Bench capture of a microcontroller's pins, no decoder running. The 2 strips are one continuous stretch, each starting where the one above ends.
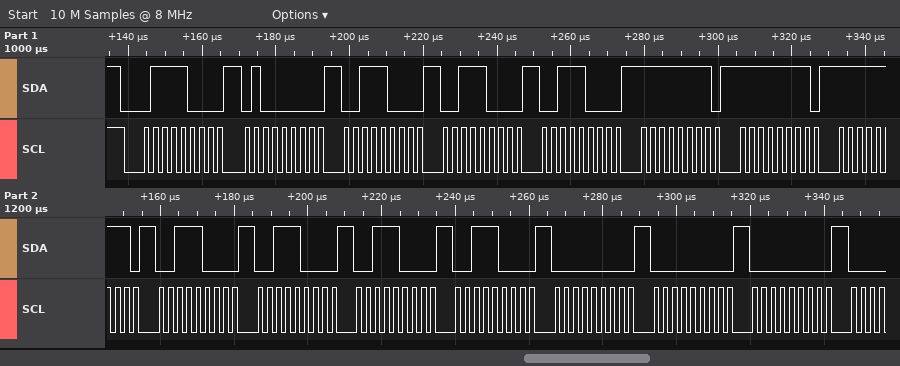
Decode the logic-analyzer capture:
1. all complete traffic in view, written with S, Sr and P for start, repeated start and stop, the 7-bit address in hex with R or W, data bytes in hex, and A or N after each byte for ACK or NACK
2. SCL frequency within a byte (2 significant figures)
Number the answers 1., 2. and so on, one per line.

1. S 3CW A 40 A 38 A 38 A 38 A FF A FF A FF A 38 A 38 A 38 A 38 A 00 A 00 A 00 A
2. 400 kHz
